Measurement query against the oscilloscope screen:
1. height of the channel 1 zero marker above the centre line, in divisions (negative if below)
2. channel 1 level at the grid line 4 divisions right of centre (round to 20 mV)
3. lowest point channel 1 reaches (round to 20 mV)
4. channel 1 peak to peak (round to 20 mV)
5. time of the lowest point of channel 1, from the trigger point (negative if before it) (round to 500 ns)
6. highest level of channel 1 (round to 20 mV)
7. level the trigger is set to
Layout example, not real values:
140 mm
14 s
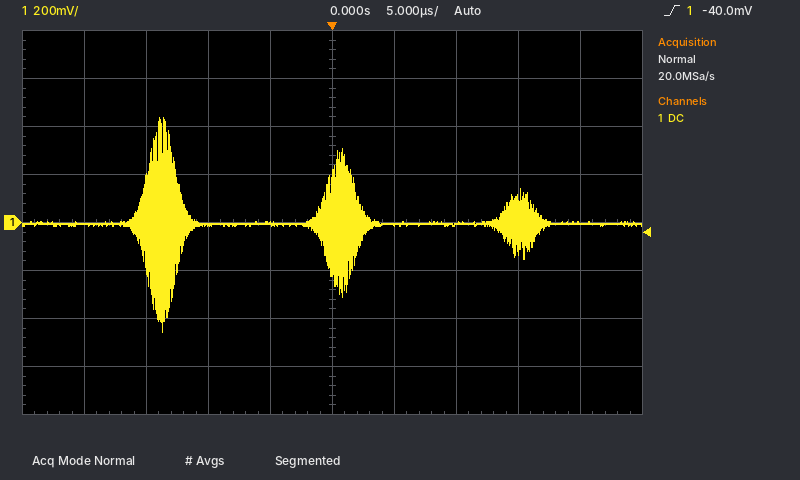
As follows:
0.0 div
0 mV
-460 mV
900 mV
-13.5 µs
440 mV
-40.0 mV
